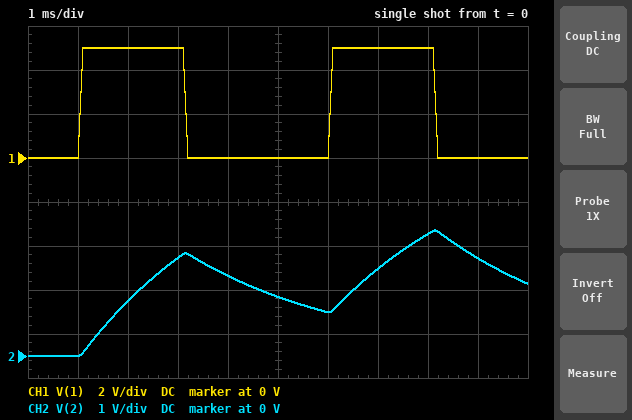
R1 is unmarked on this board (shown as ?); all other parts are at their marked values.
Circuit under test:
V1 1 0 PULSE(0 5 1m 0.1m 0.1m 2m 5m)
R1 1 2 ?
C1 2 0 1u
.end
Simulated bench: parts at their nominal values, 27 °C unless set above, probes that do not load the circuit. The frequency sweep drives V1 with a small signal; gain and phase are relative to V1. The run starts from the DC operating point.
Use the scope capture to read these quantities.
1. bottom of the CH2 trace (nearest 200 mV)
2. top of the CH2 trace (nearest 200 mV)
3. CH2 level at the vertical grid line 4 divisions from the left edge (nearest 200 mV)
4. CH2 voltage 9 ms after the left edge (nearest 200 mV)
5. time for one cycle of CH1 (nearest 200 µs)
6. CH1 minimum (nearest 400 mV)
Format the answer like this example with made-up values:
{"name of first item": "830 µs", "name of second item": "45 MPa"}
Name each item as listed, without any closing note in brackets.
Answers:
{"bottom of the CH2 trace": "0 V", "top of the CH2 trace": "2.8 V", "CH2 level at the vertical grid line 4 divisions from the left edge": "1.8 V", "CH2 voltage 9 ms after the left edge": "2.2 V", "time for one cycle of CH1": "5.0 ms", "CH1 minimum": "0 V"}
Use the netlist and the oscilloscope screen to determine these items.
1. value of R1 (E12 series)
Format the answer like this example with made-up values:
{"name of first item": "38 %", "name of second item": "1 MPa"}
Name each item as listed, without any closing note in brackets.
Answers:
{"value of R1": "3.3 kΩ"}
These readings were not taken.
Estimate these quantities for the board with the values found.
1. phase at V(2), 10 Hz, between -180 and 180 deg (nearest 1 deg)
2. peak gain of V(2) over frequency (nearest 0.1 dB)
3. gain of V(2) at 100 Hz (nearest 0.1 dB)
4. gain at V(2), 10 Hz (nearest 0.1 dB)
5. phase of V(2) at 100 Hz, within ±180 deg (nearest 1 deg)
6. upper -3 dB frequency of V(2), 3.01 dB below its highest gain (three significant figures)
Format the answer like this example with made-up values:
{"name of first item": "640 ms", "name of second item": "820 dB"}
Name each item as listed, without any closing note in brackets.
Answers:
{"phase at V(2), 10 Hz, between -180 and 180 deg": "-12 deg", "peak gain of V(2) over frequency": "0 dB", "gain of V(2) at 100 Hz": "-7.2 dB", "gain at V(2), 10 Hz": "-0.2 dB", "phase of V(2) at 100 Hz, within ±180 deg": "-64 deg", "upper -3 dB frequency of V(2), 3.01 dB below its highest gain": "48.2 Hz"}
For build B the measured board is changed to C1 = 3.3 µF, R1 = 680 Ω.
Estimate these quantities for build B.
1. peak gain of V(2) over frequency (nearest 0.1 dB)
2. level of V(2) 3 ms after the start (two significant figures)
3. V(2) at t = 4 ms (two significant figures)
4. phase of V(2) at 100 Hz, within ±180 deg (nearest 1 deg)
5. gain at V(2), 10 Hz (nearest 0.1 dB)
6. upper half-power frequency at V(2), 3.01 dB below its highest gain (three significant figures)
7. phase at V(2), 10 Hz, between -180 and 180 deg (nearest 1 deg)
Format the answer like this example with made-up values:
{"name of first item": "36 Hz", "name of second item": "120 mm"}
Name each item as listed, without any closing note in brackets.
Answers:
{"peak gain of V(2) over frequency": "0 dB", "level of V(2) 3 ms after the start": "2.9 V", "V(2) at t = 4 ms": "2.1 V", "phase of V(2) at 100 Hz, within ±180 deg": "-55 deg", "gain at V(2), 10 Hz": "-0.1 dB", "upper half-power frequency at V(2), 3.01 dB below its highest gain": "70.9 Hz", "phase at V(2), 10 Hz, between -180 and 180 deg": "-8 deg"}
